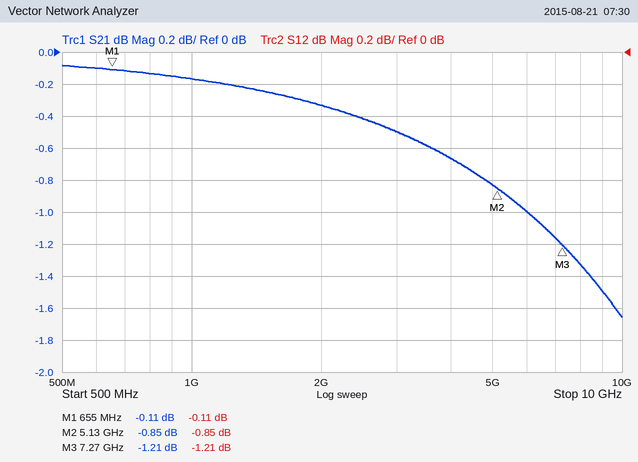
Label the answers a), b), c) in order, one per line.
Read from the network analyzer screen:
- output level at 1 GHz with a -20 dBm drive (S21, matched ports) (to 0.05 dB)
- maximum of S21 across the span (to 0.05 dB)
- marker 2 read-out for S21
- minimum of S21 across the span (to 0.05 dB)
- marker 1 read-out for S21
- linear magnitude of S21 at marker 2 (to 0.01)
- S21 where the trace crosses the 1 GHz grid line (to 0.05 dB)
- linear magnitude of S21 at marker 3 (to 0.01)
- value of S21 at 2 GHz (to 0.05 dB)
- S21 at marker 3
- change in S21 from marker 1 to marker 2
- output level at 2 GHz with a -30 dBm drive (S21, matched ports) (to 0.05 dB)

a) -20.15 dBm
b) -0.10 dB
c) -0.85 dB
d) -1.65 dB
e) -0.11 dB
f) 0.91
g) -0.15 dB
h) 0.87
i) -0.35 dB
j) -1.21 dB
k) -0.74 dB
l) -30.35 dBm
